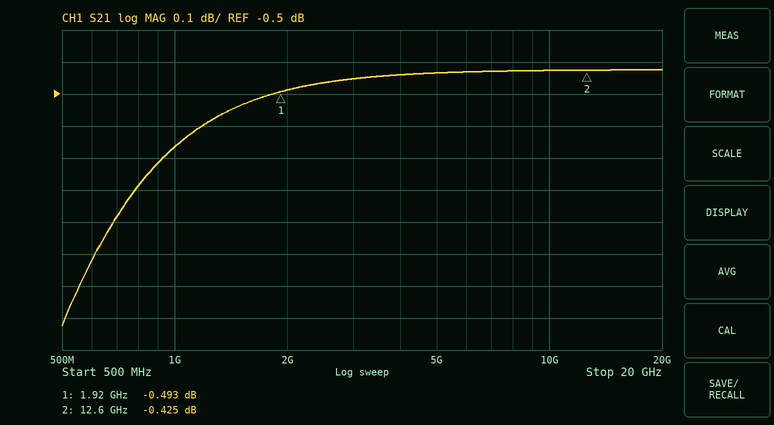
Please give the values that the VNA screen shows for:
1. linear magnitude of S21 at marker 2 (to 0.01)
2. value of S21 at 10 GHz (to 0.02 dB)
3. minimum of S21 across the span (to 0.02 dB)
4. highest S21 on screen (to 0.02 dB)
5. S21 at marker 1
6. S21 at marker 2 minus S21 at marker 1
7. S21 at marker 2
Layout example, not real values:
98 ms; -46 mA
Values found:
0.95; -0.42 dB; -1.22 dB; -0.42 dB; -0.493 dB; 0.068 dB; -0.425 dB
